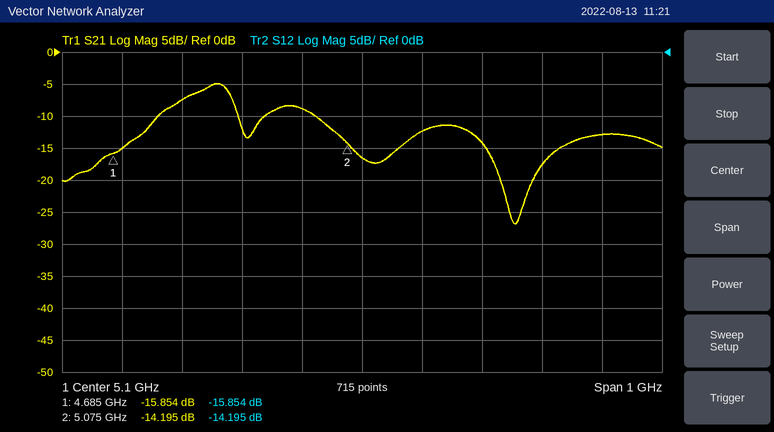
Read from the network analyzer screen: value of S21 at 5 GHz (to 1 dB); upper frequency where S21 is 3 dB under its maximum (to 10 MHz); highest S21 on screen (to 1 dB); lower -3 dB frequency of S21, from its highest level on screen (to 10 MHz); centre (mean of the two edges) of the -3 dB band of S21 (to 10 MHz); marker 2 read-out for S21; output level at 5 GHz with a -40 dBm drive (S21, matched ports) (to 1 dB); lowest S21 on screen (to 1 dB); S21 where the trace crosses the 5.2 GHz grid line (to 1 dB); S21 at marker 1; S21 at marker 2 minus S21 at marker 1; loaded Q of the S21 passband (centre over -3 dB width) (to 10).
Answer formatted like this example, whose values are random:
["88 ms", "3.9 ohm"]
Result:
["-9 dB", "4.89 GHz", "-5 dB", "4.79 GHz", "4.84 GHz", "-14.195 dB", "-49 dBm", "-27 dB", "-12 dB", "-15.854 dB", "1.659 dB", "50"]
